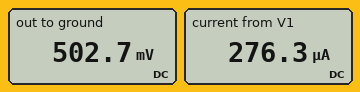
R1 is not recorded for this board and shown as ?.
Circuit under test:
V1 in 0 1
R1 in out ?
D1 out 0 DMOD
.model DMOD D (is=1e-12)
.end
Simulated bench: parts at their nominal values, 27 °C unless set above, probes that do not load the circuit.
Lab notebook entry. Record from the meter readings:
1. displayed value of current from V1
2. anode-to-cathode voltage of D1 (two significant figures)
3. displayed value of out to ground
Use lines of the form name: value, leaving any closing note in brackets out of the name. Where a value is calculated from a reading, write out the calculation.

displayed value of current from V1: 276.3 µA
anode-to-cathode voltage of D1: 502.7 mV = 500 mV
displayed value of out to ground: 502.7 mV
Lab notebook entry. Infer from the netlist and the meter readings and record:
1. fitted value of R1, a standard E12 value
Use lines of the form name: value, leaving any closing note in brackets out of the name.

fitted value of R1, a standard E12 value: 1.8 kΩ
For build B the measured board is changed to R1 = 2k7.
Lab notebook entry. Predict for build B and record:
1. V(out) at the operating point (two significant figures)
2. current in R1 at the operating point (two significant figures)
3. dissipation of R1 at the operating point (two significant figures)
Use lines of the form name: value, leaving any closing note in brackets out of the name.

V(out) at the operating point: 490 mV
current in R1 at the operating point: 190 µA
dissipation of R1 at the operating point: 95 µW
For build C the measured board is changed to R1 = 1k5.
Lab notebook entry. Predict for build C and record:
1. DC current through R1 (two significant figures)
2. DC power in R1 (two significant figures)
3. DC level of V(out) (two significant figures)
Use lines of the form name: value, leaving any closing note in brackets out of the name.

DC current through R1: 330 µA
DC power in R1: 160 µW
DC level of V(out): 510 mV
